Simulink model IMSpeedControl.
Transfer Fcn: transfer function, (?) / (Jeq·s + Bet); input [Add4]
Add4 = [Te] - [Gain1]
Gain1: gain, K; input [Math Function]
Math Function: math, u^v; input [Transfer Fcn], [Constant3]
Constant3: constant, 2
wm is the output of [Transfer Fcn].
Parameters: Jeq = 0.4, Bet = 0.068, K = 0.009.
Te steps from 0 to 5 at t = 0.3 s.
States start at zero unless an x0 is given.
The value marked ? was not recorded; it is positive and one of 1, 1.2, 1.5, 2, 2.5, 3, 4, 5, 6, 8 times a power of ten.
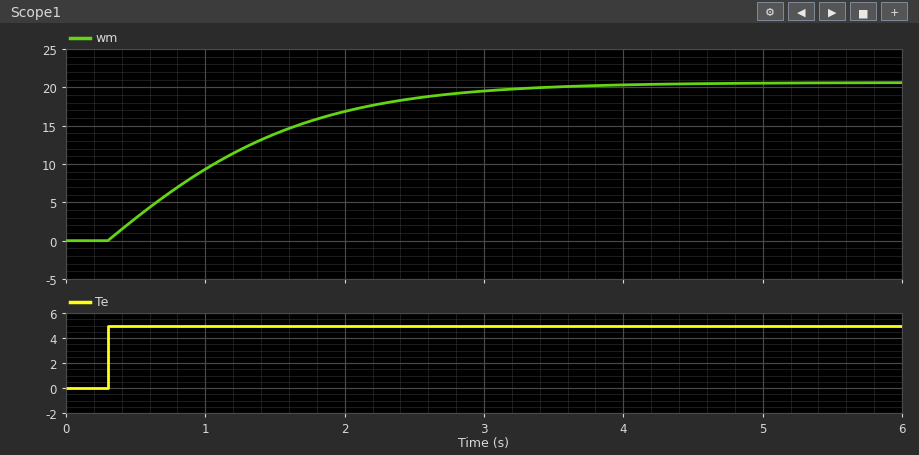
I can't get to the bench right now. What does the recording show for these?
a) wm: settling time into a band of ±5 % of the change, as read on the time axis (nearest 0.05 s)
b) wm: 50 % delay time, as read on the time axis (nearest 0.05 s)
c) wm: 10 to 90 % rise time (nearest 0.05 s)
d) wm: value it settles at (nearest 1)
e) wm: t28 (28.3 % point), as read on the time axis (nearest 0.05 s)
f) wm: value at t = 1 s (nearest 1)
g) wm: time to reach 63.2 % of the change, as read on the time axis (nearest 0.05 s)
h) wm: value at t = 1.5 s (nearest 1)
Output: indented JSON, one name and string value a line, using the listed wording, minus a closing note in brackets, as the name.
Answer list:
{
  "wm: settling time into a band of ±5 % of the change, as read on the time axis": "3.05 s",
  "wm: 50 % delay time, as read on the time axis": "1.10 s",
  "wm: 10 to 90 % rise time": "2.05 s",
  "wm: value it settles at": "21",
  "wm: t28 (28.3 % point), as read on the time axis": "0.70 s",
  "wm: value at t = 1 s": "9",
  "wm: time to reach 63.2 % of the change, as read on the time axis": "1.40 s",
  "wm: value at t = 1.5 s": "14"
}
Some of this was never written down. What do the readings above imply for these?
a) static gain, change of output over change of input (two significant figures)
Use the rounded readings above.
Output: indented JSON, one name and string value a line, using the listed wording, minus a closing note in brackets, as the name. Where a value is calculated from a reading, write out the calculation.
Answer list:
{
  "static gain, change of output over change of input": "(21 - 0) / (5 - 0) = 4.2"
}
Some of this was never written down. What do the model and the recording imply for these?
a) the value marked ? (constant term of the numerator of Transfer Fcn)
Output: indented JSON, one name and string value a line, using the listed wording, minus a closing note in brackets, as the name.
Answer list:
{
  "the value marked ?": "1.2"
}
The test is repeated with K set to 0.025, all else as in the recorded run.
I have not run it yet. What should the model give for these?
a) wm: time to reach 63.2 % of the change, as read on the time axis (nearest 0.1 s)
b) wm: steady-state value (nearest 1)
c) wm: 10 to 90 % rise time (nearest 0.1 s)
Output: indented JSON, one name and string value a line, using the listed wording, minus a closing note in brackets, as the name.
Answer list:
{
  "wm: time to reach 63.2 % of the change, as read on the time axis": "1.0 s",
  "wm: steady-state value": "13",
  "wm: 10 to 90 % rise time": "1.3 s"
}
